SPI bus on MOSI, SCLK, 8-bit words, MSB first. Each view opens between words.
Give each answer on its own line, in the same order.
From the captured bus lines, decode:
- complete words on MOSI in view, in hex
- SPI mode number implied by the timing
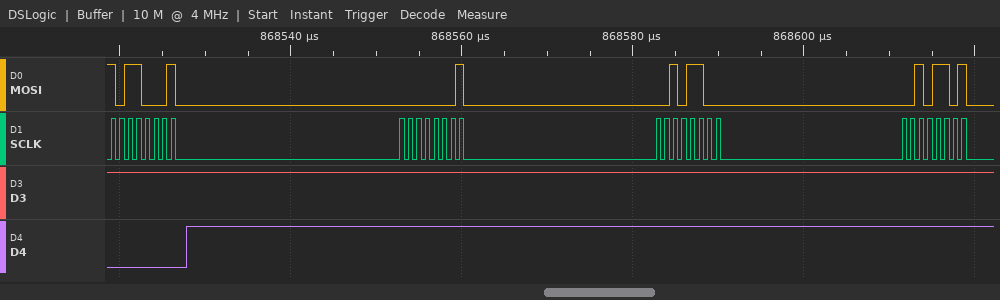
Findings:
B1, 01, 2C, 2D
0
